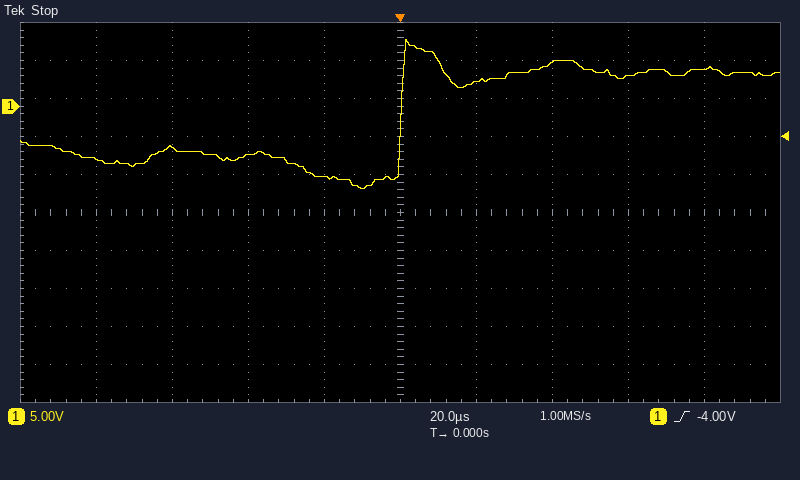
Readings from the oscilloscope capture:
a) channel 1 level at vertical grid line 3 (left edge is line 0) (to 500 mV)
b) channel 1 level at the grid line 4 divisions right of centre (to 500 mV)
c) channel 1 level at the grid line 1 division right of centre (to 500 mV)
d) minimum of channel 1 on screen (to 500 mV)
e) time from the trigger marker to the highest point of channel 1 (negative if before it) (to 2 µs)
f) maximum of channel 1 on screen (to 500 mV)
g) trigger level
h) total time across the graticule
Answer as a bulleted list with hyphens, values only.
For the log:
- -6.5 V
- 5.0 V
- 3.0 V
- -11.0 V
- +2 µs
- 9.0 V
- -4.00 V
- 200 µs
